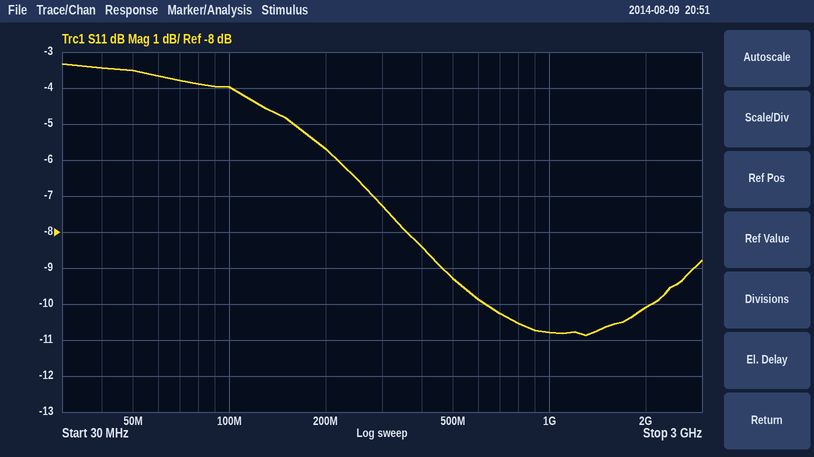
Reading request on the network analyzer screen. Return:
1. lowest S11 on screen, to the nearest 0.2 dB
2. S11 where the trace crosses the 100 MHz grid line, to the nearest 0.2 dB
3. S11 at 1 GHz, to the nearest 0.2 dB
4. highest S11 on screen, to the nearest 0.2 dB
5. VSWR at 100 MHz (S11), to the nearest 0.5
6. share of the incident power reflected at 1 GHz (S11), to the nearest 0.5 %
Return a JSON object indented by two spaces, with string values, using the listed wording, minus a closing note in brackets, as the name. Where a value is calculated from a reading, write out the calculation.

{
  "lowest S11 on screen, to the nearest 0.2 dB": "-10.8 dB",
  "S11 where the trace crosses the 100 MHz grid line, to the nearest 0.2 dB": "-4.0 dB",
  "S11 at 1 GHz, to the nearest 0.2 dB": "-10.8 dB",
  "highest S11 on screen, to the nearest 0.2 dB": "-3.4 dB",
  "VSWR at 100 MHz (S11), to the nearest 0.5": "|Γ| = 10^(-4/20) = 0.6310; VSWR = (1 + 0.6310)/(1 − 0.6310) ≈ 4.42, so 4.5 to the nearest 0.5",
  "share of the incident power reflected at 1 GHz (S11), to the nearest 0.5 %": "10^(-10.8/10) ≈ 8.32 %, so 8.5 % to the nearest 0.5 %"
}
